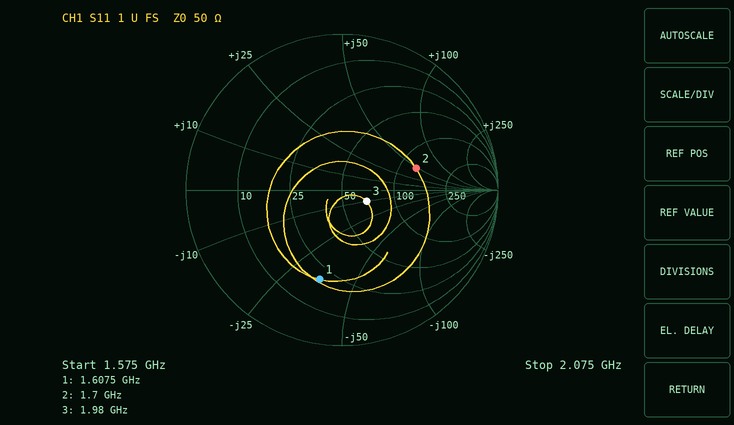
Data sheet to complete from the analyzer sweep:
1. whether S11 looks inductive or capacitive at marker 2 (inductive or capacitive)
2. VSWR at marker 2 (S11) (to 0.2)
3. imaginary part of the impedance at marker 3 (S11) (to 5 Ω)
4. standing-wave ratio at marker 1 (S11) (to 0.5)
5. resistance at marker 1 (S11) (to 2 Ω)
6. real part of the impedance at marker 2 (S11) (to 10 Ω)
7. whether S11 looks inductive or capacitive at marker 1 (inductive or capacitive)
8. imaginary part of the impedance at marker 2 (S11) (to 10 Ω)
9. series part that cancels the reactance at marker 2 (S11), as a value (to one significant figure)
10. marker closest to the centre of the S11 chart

inductive
3.0
-10 Ω
4.0
20 Ω
130 Ω
capacitive
+50 Ω
2 pF
marker 3
